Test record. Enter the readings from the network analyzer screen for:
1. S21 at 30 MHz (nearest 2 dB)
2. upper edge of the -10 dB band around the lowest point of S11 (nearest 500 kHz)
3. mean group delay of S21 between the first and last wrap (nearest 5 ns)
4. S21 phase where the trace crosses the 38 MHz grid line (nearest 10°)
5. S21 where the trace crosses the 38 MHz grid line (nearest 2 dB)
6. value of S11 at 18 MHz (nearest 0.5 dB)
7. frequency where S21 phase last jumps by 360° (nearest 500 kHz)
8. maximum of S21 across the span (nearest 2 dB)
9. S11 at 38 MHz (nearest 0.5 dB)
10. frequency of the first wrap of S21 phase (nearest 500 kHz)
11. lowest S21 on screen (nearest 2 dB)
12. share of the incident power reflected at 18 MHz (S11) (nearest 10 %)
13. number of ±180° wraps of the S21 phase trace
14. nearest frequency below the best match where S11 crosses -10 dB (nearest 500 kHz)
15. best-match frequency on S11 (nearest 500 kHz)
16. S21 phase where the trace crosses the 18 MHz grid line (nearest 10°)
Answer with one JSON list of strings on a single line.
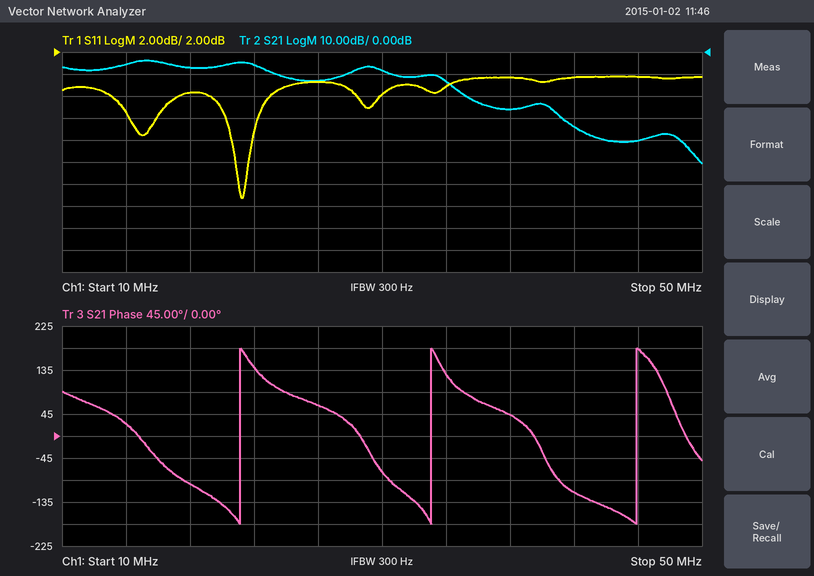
["-8 dB", "21.5 MHz", "80 ns", "40°", "-26 dB", "-1.5 dB", "46.0 MHz", "-4 dB", "-0.5 dB", "21.0 MHz", "-50 dB", "70 %", "3", "21.0 MHz", "21.0 MHz", "-100°"]
